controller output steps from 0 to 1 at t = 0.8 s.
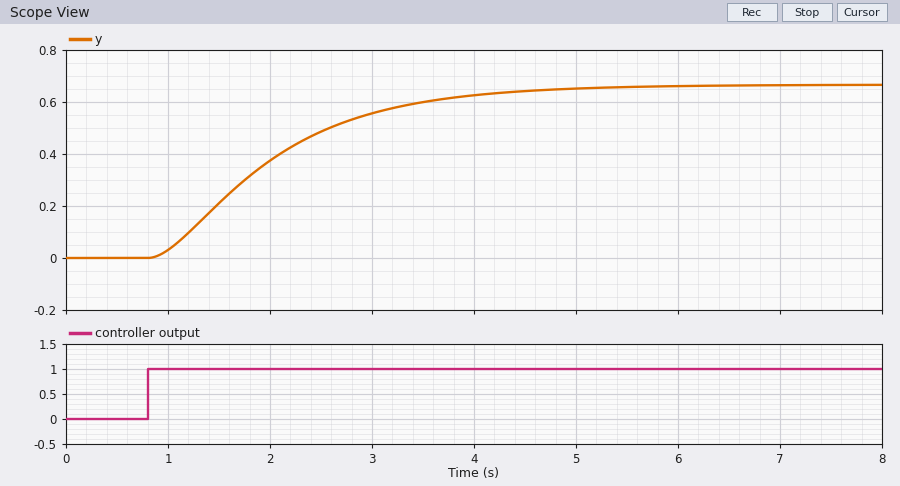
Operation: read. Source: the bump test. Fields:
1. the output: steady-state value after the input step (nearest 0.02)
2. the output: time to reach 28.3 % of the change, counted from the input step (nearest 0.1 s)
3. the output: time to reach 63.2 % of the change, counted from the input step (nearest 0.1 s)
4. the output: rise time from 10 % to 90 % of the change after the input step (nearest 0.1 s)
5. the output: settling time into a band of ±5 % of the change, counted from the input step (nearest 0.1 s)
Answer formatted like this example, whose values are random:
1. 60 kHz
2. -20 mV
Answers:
1. 0.66
2. 0.6 s
3. 1.4 s
4. 2.4 s
5. 3.4 s
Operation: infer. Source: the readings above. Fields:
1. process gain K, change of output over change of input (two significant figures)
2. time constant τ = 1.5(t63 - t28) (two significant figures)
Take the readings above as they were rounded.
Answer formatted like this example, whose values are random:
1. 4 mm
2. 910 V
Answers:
1. 0.66
2. 1.2 s
